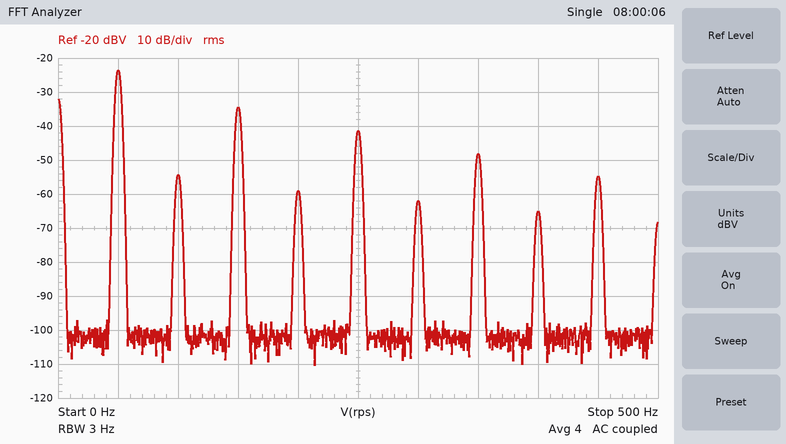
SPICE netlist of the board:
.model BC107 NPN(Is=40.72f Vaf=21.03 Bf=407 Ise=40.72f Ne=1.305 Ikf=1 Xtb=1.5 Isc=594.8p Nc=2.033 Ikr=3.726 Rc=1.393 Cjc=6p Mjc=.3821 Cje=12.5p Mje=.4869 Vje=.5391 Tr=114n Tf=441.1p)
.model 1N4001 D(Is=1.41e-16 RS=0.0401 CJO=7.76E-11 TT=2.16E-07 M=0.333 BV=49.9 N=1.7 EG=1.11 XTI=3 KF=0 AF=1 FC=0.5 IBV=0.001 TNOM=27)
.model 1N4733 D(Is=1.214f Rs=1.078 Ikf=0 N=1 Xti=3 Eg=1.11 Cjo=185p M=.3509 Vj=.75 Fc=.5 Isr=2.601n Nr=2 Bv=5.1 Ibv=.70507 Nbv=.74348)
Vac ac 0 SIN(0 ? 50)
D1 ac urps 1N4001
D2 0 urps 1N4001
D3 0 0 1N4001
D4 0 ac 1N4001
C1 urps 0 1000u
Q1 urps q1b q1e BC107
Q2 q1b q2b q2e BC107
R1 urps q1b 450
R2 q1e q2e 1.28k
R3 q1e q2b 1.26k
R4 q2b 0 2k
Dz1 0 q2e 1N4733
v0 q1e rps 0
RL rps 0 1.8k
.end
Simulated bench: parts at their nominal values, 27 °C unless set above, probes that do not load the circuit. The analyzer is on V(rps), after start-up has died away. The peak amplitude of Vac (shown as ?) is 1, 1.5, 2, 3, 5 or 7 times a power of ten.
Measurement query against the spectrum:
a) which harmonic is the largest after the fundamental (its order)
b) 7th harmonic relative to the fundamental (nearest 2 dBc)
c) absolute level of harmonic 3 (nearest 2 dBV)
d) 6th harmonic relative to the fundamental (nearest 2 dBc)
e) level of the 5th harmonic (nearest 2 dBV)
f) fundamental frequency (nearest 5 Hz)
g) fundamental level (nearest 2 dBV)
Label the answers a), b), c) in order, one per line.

a) 3
b) -24 dBc
c) -34 dBV
d) -38 dBc
e) -42 dBV
f) 50 Hz
g) -24 dBV
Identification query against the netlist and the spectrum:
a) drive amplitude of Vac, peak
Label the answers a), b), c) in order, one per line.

a) 30 V
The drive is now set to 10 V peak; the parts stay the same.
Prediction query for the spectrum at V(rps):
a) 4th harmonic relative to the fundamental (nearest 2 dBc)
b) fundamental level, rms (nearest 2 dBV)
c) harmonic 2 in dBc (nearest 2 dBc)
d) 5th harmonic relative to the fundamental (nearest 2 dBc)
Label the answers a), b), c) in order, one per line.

a) -12 dBc
b) -28 dBV
c) -6 dBc
d) -14 dBc
